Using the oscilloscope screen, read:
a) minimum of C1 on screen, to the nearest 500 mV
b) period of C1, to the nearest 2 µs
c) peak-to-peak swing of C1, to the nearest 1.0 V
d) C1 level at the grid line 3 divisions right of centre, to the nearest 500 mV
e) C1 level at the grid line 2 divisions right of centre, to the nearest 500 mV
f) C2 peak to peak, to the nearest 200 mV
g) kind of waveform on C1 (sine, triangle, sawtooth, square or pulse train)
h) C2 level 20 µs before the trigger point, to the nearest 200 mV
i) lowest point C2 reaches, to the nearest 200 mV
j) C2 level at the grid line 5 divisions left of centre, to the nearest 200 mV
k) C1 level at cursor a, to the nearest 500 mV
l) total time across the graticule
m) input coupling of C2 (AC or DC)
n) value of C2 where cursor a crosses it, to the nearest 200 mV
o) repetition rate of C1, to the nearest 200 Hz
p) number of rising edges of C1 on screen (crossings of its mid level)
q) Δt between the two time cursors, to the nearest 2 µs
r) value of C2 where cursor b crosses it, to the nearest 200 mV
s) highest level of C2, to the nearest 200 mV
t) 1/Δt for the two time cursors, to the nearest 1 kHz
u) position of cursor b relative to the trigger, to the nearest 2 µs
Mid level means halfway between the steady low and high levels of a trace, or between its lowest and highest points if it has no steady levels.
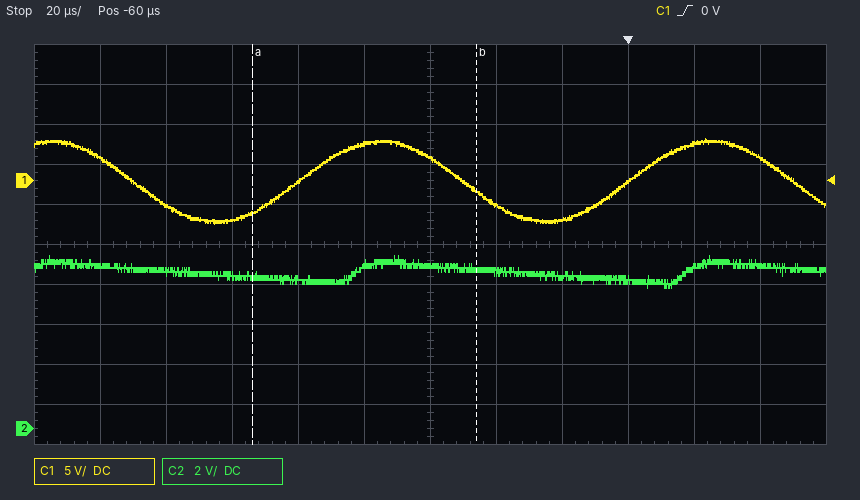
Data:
-5.5 V
100 µs
11.0 V
0.0 V
-5.0 V
1.6 V
sine
7.6 V
7.0 V
8.2 V
-4.0 V
240 µs
DC
7.6 V
10.0 kHz
2
68 µs
8.0 V
8.6 V
15 kHz
-46 µs
